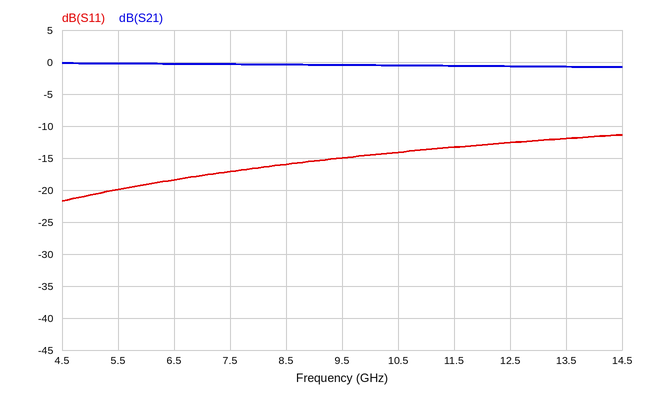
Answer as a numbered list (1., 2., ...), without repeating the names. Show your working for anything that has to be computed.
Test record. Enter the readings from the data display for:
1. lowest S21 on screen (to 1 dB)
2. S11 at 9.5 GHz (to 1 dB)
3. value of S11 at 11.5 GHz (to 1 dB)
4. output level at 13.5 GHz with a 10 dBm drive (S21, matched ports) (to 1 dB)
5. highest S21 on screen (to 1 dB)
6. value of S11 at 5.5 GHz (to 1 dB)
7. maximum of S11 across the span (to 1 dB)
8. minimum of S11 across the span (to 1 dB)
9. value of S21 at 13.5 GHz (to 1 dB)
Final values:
1. -1 dB
2. -15 dB
3. -13 dB
4. 10 dBm + (-1 dB) = 9 dBm
5. 0 dB
6. -20 dB
7. -11 dB
8. -22 dB
9. -1 dB
